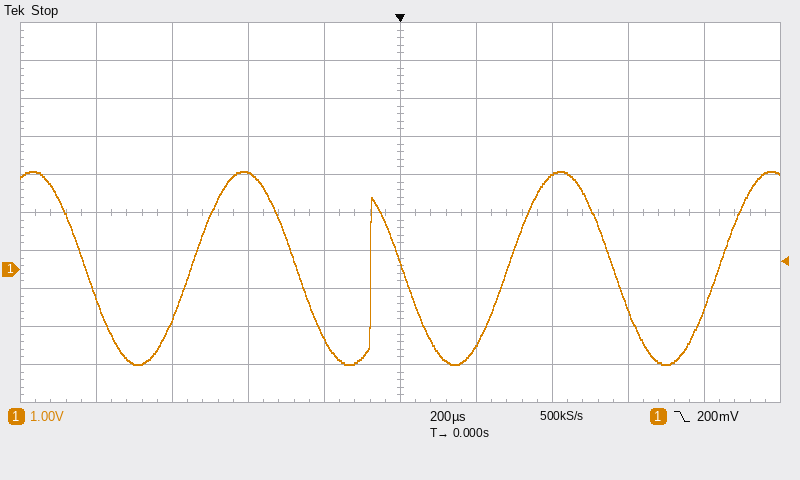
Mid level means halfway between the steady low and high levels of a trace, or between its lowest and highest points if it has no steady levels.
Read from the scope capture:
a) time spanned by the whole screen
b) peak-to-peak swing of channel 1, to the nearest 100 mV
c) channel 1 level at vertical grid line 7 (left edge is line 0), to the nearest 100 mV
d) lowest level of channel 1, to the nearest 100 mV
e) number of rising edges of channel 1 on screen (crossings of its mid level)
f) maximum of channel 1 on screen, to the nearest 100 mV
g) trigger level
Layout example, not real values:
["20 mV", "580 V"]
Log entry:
["2 ms", "5.1 V", "2.5 V", "-2.5 V", "4", "2.6 V", "200 mV"]
